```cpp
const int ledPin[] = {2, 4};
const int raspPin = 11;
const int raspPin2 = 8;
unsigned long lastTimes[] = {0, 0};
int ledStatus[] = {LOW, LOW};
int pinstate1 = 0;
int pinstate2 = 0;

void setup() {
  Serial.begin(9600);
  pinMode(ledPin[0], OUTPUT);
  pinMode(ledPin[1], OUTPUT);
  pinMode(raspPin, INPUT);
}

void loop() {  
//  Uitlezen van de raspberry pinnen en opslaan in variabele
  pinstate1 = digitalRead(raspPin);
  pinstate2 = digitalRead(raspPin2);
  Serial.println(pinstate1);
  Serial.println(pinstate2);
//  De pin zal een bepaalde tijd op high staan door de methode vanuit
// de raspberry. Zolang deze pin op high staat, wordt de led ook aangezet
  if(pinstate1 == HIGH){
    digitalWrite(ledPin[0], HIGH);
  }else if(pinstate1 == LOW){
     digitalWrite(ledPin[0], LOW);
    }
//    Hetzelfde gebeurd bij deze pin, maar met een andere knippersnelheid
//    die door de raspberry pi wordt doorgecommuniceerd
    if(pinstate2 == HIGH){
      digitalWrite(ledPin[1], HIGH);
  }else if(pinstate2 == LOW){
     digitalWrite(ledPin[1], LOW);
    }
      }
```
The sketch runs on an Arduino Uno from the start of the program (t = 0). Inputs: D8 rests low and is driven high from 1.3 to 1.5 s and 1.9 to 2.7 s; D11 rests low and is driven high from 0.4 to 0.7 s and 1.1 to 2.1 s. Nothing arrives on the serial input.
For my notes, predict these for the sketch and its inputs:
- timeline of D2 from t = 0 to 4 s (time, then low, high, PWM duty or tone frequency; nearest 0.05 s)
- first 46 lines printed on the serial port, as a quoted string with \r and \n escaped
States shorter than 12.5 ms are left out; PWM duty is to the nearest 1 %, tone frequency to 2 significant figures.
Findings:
0 s low; 0.4 s high; 0.7 s low; 1.1 s high; 2.1 s low
"0\r\n0\r\n0\r\n0\r\n0\r\n0\r\n0\r\n0\r\n0\r\n0\r\n0\r\n0\r\n0\r\n0\r\n0\r\n0\r\n0\r\n0\r\n0\r\n0\r\n0\r\n0\r\n0\r\n0\r\n0\r\n0\r\n0\r\n0\r\n0\r\n0\r\n0\r\n0\r\n0\r\n0\r\n0\r\n0\r\n0\r\n0\r\n0\r\n0\r\n0\r\n0\r\n0\r\n0\r\n0\r\n0\r\n"
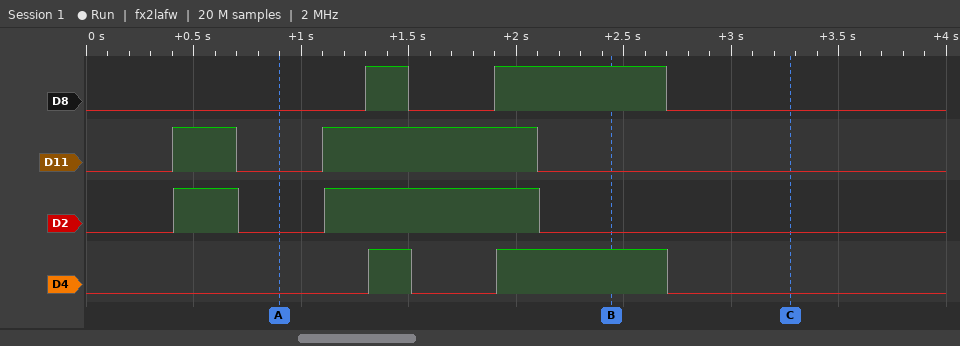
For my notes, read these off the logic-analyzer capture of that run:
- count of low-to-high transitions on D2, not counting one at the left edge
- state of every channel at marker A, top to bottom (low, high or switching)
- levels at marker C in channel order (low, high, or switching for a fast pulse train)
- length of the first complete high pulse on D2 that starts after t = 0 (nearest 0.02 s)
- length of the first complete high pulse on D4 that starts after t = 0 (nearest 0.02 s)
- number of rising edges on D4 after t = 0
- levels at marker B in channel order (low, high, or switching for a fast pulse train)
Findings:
2
D8 low, D11 low, D2 low, D4 low
D8 low, D11 low, D2 low, D4 low
0.30 s
0.20 s
2
D8 high, D11 low, D2 low, D4 high
